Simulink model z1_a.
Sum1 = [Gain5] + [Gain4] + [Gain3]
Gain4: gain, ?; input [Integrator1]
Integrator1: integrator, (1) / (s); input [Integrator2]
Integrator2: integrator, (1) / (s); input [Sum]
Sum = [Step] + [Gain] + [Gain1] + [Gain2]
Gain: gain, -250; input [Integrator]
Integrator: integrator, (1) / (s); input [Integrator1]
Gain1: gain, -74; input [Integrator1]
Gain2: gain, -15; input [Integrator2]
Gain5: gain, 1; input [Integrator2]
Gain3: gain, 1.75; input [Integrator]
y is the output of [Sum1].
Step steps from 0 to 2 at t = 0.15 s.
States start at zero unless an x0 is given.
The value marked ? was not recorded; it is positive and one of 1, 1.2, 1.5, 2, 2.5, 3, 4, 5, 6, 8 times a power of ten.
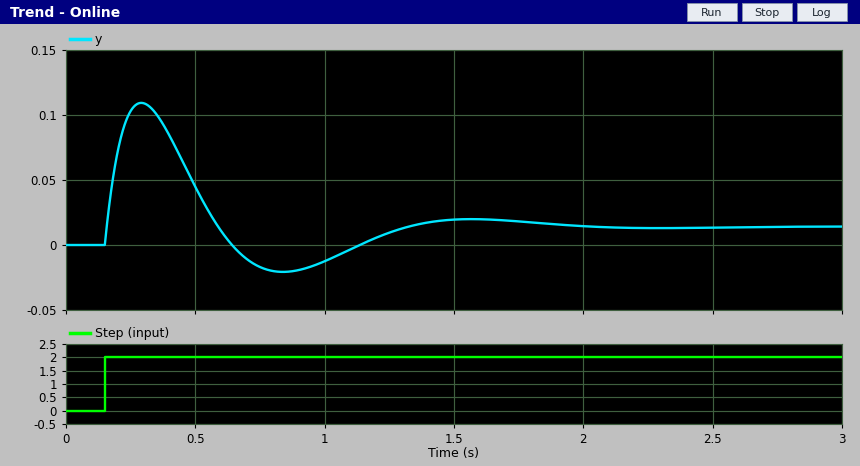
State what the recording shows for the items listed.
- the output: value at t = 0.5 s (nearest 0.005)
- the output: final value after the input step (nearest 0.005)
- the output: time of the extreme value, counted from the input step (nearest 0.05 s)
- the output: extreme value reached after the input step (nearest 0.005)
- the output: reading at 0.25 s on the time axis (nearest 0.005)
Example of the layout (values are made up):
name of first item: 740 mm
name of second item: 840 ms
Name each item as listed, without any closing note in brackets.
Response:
the output: value at t = 0.5 s: 0.045
the output: final value after the input step: 0.015
the output: time of the extreme value, counted from the input step: 0.15 s
the output: extreme value reached after the input step: 0.110
the output: reading at 0.25 s on the time axis: 0.105
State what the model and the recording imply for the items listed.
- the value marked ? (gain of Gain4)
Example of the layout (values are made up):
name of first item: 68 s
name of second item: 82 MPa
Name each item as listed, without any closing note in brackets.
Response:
the value marked ?: 2
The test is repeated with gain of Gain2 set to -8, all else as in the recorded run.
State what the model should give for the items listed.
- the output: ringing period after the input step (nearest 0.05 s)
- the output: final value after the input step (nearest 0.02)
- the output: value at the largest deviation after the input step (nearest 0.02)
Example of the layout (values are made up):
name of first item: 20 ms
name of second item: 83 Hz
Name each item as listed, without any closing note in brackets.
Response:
the output: ringing period after the input step: 0.85 s
the output: final value after the input step: 0.02
the output: value at the largest deviation after the input step: 0.16
